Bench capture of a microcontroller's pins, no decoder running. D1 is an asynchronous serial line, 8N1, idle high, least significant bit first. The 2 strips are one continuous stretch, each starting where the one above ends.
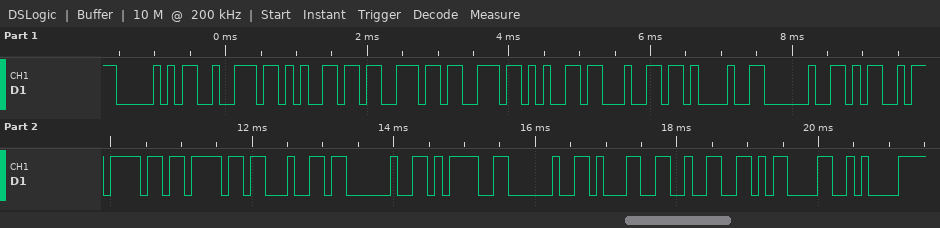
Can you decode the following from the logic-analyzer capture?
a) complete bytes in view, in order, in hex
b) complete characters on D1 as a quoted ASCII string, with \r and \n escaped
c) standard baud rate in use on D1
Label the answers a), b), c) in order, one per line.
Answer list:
a) 50 72 65 73 73 65 64 21 20 4D 6F 6F 64 20 3D 20 31 32 0D 0A
b) "Pressed! Mood = 12\r\n"
c) 9600 baud
